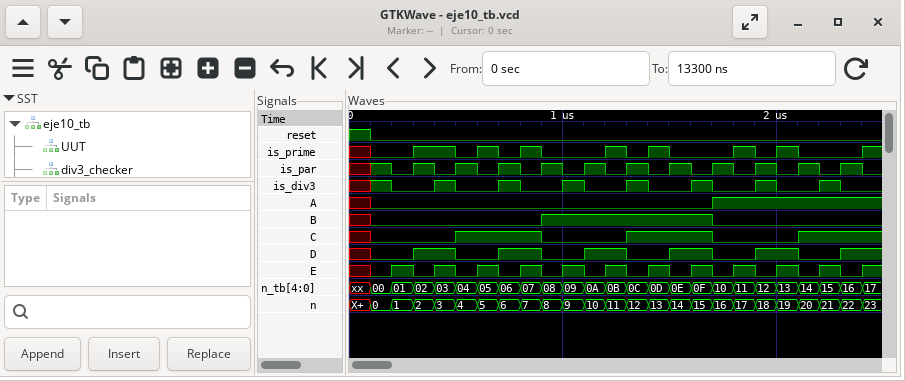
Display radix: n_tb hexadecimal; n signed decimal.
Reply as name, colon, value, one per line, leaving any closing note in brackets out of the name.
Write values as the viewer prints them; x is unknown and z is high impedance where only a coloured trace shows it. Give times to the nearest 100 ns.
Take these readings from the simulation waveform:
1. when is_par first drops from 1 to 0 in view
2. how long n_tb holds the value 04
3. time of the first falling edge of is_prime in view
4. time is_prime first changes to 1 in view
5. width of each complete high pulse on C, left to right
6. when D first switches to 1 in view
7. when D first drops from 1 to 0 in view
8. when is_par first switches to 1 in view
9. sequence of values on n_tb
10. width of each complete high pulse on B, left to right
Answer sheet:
when is_par first drops from 1 to 0 in view: 200 ns
how long n_tb holds the value 04: 100 ns
time of the first falling edge of is_prime in view: 500 ns
time is_prime first changes to 1 in view: 300 ns
width of each complete high pulse on C, left to right: 400 ns, 400 ns
when D first switches to 1 in view: 300 ns
when D first drops from 1 to 0 in view: 500 ns
when is_par first switches to 1 in view: 100 ns
sequence of values on n_tb: xx, 00, 01, 02, 03, 04, 05, 06, 07, 08, 09, 0A, 0B, 0C, 0D, 0E, 0F, 10, 11, 12, 13, 14, 15, 16, 17
width of each complete high pulse on B, left to right: 800 ns
